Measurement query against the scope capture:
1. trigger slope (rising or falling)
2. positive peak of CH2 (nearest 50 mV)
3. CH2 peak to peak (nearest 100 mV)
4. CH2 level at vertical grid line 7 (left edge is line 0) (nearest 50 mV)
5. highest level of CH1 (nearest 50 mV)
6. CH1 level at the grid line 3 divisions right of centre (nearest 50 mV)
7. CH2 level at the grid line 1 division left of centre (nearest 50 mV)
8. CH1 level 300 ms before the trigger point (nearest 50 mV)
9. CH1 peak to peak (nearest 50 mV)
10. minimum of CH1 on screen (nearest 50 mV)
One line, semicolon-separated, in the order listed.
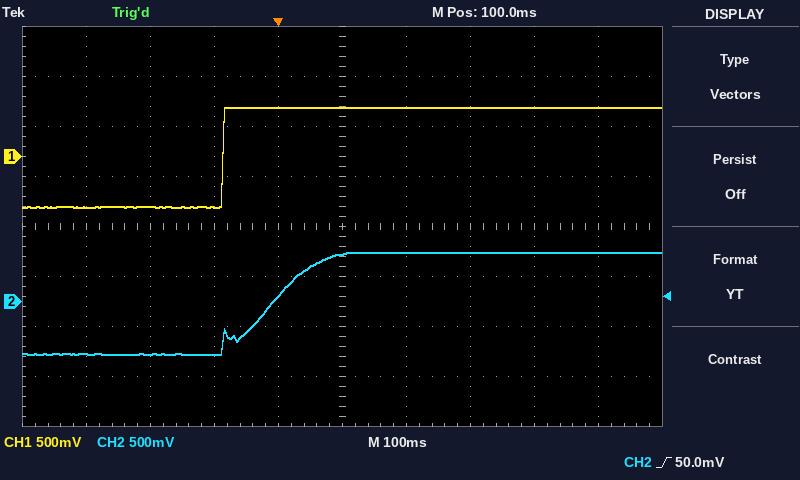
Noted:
rising; 500 mV; 1.00 V; 500 mV; 500 mV; 500 mV; 50 mV; -500 mV; 1.00 V; -500 mV
